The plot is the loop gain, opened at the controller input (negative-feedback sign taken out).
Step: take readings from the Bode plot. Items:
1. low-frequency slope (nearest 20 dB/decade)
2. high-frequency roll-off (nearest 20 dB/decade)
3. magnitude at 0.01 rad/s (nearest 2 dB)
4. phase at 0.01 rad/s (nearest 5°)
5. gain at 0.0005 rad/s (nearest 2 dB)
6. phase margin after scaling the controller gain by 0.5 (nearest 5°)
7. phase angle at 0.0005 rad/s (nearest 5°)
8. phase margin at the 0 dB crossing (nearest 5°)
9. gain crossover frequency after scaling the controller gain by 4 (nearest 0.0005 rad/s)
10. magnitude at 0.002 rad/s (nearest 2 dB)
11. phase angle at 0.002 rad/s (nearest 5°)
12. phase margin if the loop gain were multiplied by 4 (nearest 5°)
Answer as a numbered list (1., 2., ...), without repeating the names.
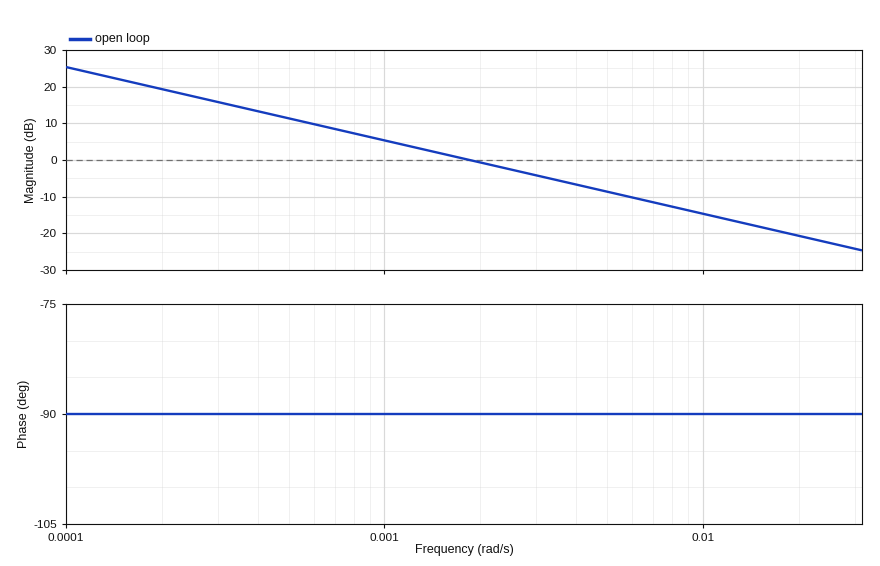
1. -20 dB/decade
2. -20 dB/decade
3. -14 dB
4. -90°
5. 12 dB
6. 90°
7. -90°
8. 90°
9. 0.0075 rad/s
10. 0 dB
11. -90°
12. 90°
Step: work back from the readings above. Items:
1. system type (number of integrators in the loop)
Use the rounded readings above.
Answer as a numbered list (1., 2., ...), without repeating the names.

1. 1
